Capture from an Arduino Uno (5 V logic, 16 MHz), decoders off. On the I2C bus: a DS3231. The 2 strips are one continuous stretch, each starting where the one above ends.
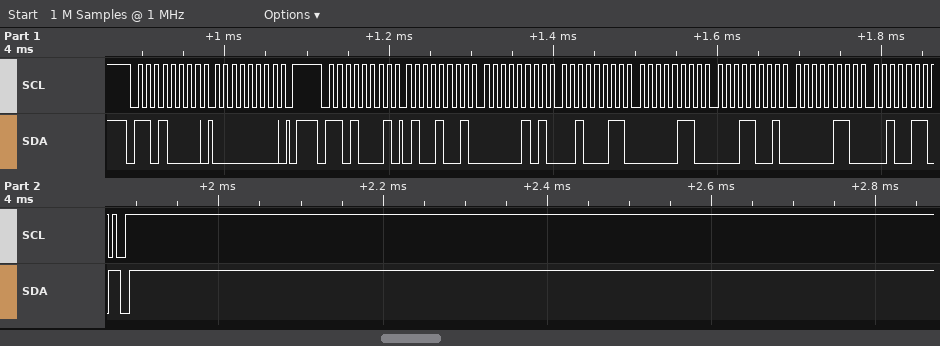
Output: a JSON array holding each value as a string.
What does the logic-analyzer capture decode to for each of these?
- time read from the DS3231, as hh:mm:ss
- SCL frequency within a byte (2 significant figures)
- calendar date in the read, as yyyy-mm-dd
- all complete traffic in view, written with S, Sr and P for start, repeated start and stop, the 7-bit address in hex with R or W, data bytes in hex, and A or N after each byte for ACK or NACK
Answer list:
["23:05:49", "100 kHz", "2026-06-19", "S 68W A 00 A P S 68R A 49 A 05 A 23 A 06 A 19 A 06 A 26 N P"]
